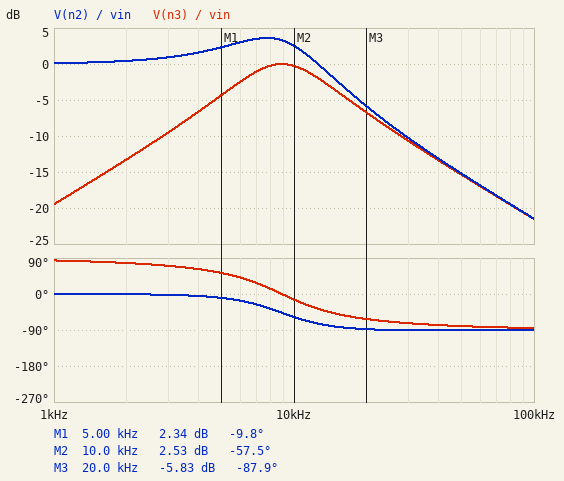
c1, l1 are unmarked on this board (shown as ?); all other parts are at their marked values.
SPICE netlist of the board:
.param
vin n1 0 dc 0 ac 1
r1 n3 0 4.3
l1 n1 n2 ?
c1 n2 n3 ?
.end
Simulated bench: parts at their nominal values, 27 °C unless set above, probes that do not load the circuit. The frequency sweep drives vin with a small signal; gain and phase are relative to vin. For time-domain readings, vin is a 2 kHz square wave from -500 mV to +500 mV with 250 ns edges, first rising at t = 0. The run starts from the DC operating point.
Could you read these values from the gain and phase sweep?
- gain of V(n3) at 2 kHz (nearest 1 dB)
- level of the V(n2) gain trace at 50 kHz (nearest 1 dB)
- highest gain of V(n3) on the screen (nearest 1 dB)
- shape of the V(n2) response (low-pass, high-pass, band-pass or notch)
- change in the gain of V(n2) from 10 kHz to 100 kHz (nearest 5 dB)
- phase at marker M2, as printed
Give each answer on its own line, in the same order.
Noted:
-13 dB
-15 dB
0 dB
low-pass
-25 dB
-57.5 deg
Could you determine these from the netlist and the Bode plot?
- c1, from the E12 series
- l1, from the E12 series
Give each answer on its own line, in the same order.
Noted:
3.9 µF
82 µH
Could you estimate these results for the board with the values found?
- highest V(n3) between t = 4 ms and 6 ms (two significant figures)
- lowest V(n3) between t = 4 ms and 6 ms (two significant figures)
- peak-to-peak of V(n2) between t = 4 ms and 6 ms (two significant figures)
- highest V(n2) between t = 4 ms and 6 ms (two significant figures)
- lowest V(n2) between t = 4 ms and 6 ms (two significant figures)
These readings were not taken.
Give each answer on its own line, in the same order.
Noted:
530 mV
-530 mV
1.6 V
820 mV
-820 mV
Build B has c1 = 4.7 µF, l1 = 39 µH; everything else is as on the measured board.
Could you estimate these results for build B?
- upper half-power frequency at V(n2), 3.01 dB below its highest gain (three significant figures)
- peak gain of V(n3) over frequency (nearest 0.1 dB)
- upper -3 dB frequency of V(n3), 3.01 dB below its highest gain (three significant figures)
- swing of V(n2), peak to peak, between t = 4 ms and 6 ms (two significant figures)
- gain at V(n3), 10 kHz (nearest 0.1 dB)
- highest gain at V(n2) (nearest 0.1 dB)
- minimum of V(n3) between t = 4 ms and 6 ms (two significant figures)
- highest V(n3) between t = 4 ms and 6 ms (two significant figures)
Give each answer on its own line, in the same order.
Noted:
19.4 kHz
0 dB
23.4 kHz
1.4 V
-0.2 dB
1.9 dB
-660 mV
660 mV
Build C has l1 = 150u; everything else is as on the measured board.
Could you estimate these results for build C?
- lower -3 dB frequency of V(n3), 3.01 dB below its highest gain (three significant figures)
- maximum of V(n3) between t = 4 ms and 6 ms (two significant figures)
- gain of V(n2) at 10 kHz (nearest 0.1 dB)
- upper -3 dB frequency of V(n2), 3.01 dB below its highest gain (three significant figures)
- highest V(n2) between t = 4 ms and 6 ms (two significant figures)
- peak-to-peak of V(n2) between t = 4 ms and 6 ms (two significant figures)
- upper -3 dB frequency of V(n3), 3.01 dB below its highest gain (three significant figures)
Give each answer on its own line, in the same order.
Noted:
4.68 kHz
460 mV
-1.3 dB
8.23 kHz
920 mV
1.8 V
9.25 kHz
